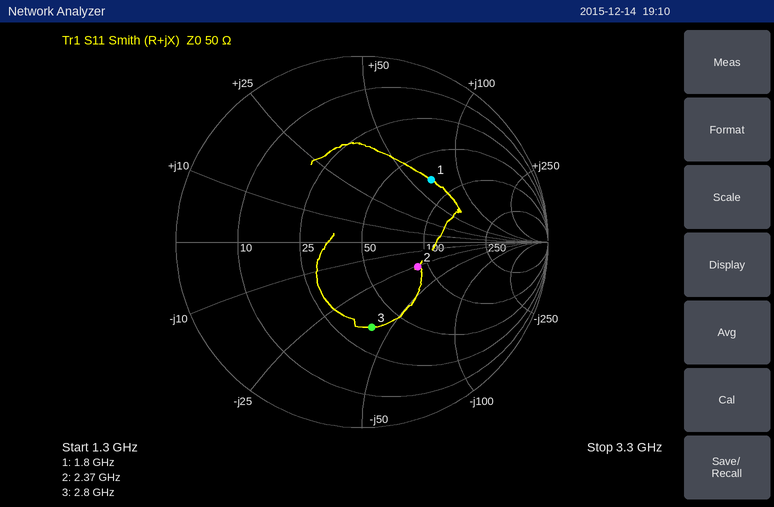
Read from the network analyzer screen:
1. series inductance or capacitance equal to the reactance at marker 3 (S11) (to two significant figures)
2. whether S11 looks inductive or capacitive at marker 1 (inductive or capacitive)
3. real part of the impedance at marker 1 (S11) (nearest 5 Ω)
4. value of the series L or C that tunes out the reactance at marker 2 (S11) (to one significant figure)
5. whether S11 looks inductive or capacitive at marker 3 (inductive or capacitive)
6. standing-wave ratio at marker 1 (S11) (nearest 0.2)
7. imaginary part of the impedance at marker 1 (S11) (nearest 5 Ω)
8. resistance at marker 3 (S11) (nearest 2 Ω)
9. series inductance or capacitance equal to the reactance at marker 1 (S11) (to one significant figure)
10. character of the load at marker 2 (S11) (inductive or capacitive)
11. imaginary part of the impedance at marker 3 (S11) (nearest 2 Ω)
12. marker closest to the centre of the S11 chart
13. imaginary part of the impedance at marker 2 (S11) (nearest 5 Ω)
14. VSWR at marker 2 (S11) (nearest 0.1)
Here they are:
1.4 pF
inductive
75 Ω
2 nH
capacitive
3.0
+65 Ω
36 Ω
6 nH
capacitive
-42 Ω
marker 2
-25 Ω
2.0
